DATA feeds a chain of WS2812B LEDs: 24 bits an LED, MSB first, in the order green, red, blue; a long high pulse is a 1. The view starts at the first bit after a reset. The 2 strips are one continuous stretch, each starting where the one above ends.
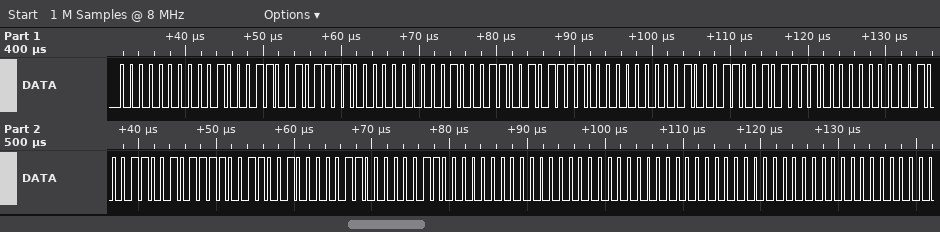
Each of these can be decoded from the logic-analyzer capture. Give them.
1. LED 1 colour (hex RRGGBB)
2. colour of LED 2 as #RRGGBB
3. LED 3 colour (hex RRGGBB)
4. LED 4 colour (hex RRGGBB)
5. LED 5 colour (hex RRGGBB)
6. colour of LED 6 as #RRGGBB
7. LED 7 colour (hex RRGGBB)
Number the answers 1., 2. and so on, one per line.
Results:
1. #23002F
2. #23002F
3. #23002F
4. #23002F
5. #0C320C
6. #000000
7. #000000
